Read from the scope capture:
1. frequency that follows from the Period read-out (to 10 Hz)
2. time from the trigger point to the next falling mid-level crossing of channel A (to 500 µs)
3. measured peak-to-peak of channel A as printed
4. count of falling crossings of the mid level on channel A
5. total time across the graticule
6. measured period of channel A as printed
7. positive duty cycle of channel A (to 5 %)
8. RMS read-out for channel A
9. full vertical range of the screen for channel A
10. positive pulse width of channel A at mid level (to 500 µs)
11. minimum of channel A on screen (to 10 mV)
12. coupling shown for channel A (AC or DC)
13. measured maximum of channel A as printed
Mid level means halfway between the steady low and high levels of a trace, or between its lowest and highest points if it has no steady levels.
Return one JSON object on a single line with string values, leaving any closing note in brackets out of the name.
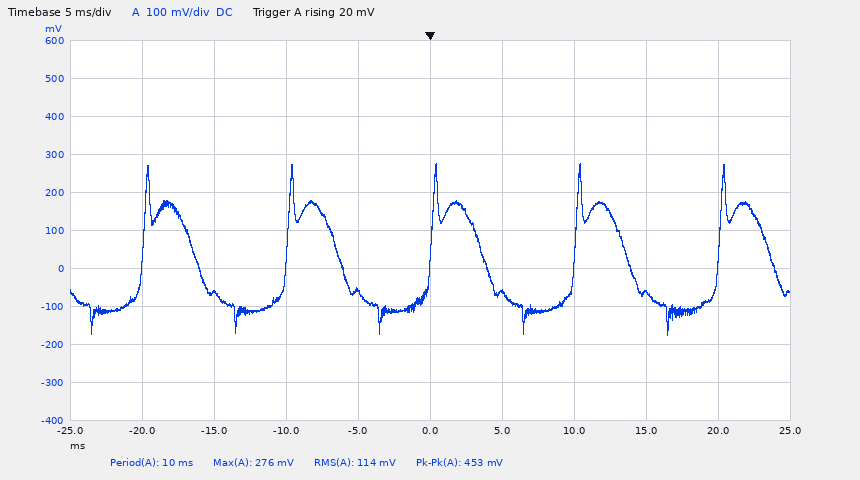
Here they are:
{"frequency that follows from the Period read-out": "100 Hz", "time from the trigger point to the next falling mid-level crossing of channel A": "3.5 ms", "measured peak-to-peak of channel A as printed": "453 mV", "count of falling crossings of the mid level on channel A": "5", "total time across the graticule": "50 ms", "measured period of channel A as printed": "10 ms", "positive duty cycle of channel A": "35 %", "RMS read-out for channel A": "114 mV", "full vertical range of the screen for channel A": "1 V", "positive pulse width of channel A at mid level": "3.5 ms", "minimum of channel A on screen": "-180 mV", "coupling shown for channel A": "DC", "measured maximum of channel A as printed": "276 mV"}
